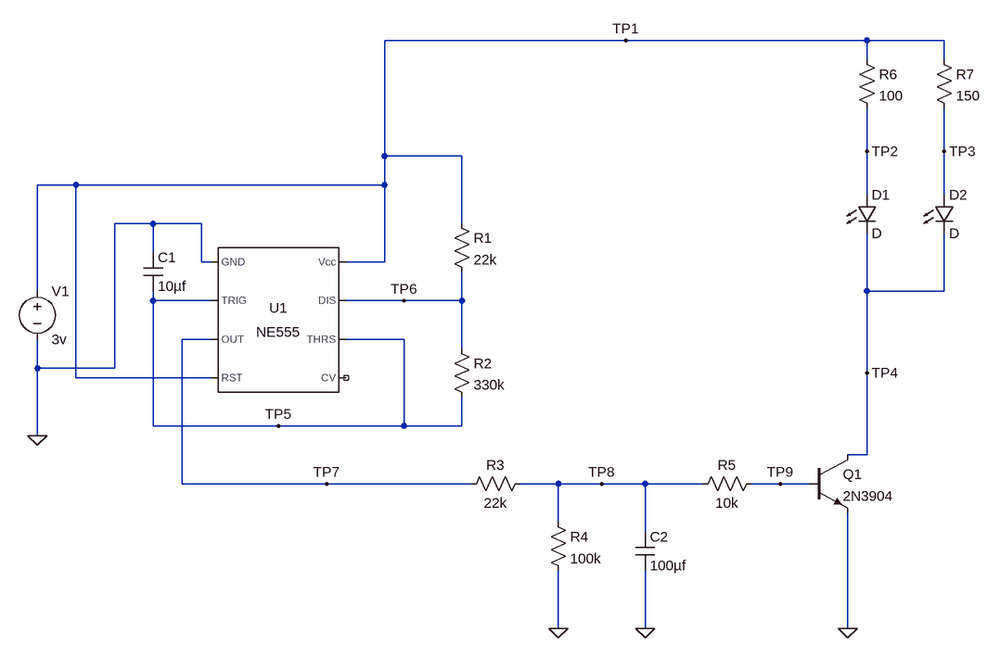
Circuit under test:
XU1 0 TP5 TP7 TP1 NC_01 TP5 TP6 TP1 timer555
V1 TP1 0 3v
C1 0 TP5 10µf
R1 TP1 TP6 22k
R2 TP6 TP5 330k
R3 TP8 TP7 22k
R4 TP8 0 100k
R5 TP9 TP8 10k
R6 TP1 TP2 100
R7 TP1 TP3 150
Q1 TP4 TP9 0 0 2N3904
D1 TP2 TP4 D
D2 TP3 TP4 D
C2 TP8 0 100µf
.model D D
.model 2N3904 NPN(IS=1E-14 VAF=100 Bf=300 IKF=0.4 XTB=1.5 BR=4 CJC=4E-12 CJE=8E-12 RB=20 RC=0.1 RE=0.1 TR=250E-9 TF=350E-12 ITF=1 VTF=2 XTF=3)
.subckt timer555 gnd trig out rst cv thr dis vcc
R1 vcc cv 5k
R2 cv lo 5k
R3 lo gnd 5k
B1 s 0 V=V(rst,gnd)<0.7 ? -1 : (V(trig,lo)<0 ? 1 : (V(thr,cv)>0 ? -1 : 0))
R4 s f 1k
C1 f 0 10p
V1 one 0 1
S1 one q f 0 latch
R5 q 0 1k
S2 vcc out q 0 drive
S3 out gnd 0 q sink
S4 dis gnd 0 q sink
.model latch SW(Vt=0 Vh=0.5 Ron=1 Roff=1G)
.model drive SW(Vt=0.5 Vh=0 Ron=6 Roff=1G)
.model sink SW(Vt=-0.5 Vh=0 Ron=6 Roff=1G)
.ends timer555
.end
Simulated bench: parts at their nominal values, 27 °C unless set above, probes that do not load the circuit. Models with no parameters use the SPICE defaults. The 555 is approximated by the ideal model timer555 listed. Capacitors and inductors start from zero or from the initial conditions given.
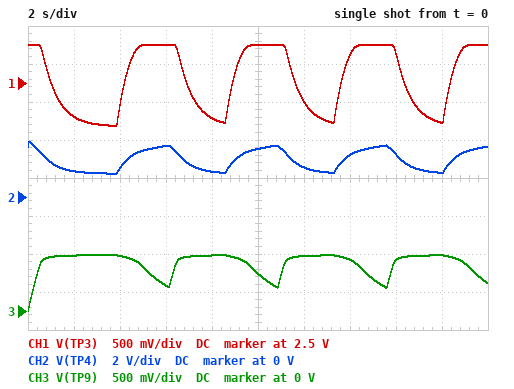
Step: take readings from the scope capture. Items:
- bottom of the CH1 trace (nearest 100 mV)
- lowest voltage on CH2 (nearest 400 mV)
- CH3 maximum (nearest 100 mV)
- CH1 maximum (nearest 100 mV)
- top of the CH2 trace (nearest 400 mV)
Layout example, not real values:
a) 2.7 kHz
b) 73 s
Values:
a) 1.9 V
b) 1.2 V
c) 700 mV
d) 3.0 V
e) 2.8 V
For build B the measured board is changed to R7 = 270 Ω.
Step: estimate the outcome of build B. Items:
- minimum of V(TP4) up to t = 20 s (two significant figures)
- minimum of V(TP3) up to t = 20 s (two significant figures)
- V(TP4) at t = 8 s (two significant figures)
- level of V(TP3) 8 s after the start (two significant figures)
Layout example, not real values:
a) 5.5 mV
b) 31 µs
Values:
a) 1.0 V
b) 1.7 V
c) 1.1 V
d) 1.8 V
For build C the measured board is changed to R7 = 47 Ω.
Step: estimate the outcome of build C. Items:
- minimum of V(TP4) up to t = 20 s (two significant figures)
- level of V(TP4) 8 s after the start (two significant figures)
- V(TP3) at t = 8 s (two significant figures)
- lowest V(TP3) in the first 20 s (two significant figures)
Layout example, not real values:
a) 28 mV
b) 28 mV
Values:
a) 1.7 V
b) 1.8 V
c) 2.5 V
d) 2.4 V
